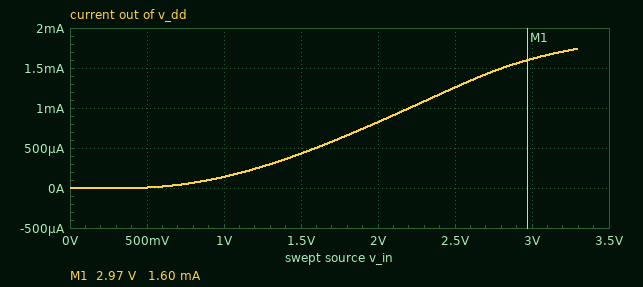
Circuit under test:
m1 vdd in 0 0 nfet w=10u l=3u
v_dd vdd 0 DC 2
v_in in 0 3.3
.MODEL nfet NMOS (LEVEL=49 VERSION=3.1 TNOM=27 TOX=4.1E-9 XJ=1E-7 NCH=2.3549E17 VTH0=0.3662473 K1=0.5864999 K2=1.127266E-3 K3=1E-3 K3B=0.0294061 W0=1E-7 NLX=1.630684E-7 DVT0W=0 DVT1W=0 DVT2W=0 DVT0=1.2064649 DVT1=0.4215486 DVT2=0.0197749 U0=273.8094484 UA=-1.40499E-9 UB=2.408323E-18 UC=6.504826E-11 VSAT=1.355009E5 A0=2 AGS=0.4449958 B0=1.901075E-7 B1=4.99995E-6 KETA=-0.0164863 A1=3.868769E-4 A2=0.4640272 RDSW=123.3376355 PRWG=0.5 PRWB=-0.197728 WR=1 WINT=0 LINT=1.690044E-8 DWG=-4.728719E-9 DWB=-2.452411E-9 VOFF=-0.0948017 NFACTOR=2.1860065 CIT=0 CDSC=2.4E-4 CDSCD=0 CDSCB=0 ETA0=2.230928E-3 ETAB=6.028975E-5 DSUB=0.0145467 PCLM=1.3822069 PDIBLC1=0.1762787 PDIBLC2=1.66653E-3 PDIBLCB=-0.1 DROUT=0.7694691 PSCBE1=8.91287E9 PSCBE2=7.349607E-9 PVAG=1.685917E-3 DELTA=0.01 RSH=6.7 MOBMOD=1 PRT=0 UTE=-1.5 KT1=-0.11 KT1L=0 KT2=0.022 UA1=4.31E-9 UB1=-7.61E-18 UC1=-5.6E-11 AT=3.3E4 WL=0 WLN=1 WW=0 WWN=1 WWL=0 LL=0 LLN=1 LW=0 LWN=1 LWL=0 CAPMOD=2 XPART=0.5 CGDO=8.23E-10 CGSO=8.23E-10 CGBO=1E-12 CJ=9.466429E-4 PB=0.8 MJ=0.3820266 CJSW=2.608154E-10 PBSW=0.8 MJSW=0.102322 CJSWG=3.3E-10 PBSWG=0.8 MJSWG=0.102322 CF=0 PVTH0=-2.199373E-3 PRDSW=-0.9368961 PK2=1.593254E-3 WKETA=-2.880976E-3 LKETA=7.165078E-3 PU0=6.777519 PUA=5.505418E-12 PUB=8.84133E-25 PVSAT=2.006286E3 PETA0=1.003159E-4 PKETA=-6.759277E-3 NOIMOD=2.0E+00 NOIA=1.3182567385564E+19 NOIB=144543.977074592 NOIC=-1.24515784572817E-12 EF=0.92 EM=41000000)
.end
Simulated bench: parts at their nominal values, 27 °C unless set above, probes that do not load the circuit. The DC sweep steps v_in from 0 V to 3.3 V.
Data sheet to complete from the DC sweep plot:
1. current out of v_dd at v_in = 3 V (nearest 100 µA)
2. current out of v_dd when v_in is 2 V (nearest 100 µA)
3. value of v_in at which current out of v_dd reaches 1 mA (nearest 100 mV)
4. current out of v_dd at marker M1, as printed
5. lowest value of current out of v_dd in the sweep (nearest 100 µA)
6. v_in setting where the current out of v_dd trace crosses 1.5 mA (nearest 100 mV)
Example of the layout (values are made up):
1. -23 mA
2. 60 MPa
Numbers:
1. 1.6 mA
2. 800 µA
3. 2.2 V
4. 1.60 mA
5. 0 A
6. 2.8 V
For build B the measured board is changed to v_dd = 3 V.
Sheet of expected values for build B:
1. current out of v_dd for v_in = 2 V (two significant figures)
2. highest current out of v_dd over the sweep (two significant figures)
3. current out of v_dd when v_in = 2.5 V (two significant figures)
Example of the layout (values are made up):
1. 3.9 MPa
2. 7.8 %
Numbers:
1. 830 µA
2. 2.0 mA
3. 1.3 mA
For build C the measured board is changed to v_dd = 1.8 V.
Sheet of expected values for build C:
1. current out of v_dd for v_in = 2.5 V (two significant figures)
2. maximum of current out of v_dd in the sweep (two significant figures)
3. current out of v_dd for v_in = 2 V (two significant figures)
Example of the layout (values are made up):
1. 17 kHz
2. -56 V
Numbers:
1. 1.2 mA
2. 1.6 mA
3. 820 µA
